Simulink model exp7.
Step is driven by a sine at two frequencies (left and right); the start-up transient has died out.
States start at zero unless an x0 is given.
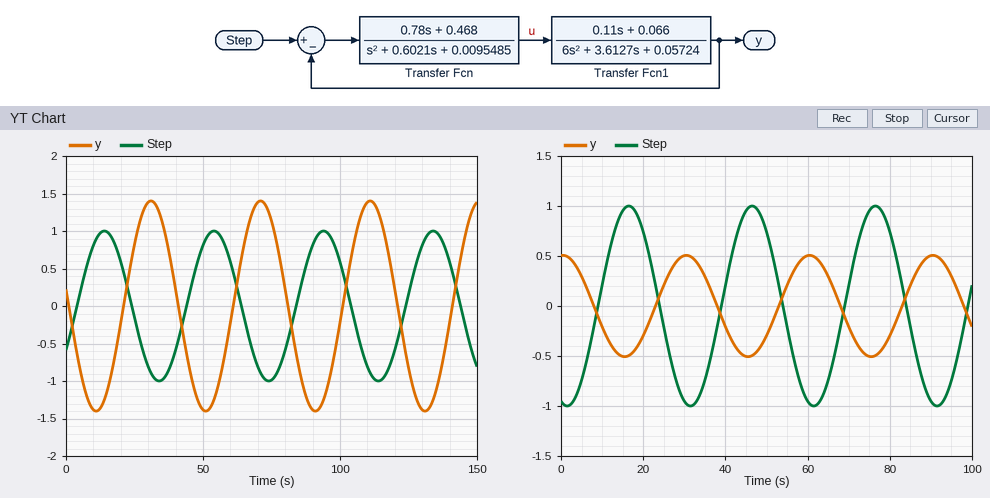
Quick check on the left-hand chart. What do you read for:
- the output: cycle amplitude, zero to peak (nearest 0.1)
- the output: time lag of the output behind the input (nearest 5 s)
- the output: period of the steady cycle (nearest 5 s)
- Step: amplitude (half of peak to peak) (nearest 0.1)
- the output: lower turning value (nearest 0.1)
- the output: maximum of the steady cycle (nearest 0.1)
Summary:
1.4
15 s
40 s
1.0
-1.4
1.4
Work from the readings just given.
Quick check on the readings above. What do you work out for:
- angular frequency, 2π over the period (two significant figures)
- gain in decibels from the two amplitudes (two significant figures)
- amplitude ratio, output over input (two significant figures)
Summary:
0.16 rad/s
2.9 dB
1.4
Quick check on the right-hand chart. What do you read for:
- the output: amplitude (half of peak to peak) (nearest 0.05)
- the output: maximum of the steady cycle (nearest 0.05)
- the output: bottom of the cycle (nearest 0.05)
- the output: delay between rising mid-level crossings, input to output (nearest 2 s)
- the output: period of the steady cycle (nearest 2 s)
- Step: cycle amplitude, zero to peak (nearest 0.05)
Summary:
0.50
0.50
-0.50
14 s
30 s
1.00
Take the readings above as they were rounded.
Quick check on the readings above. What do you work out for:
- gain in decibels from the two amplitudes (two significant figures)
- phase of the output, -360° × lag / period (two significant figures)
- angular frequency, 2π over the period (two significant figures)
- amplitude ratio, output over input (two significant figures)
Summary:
-6.0 dB
-170°
0.21 rad/s
0.50
